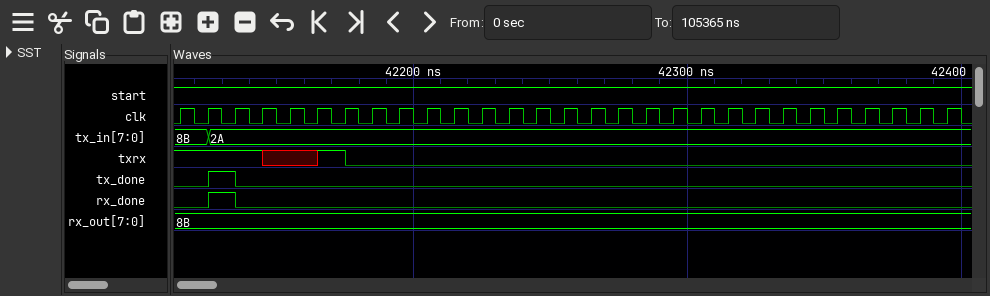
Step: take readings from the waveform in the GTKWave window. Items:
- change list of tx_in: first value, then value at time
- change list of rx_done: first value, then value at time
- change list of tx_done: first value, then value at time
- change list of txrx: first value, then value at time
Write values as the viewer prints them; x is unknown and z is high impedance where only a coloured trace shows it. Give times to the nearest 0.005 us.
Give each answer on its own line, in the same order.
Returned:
8B, 2A at 42.125 us
0, 1 at 42.125 us, 0 at 42.135 us
0, 1 at 42.125 us, 0 at 42.135 us
1, x at 42.145 us, 1 at 42.165 us, 0 at 42.175 us
